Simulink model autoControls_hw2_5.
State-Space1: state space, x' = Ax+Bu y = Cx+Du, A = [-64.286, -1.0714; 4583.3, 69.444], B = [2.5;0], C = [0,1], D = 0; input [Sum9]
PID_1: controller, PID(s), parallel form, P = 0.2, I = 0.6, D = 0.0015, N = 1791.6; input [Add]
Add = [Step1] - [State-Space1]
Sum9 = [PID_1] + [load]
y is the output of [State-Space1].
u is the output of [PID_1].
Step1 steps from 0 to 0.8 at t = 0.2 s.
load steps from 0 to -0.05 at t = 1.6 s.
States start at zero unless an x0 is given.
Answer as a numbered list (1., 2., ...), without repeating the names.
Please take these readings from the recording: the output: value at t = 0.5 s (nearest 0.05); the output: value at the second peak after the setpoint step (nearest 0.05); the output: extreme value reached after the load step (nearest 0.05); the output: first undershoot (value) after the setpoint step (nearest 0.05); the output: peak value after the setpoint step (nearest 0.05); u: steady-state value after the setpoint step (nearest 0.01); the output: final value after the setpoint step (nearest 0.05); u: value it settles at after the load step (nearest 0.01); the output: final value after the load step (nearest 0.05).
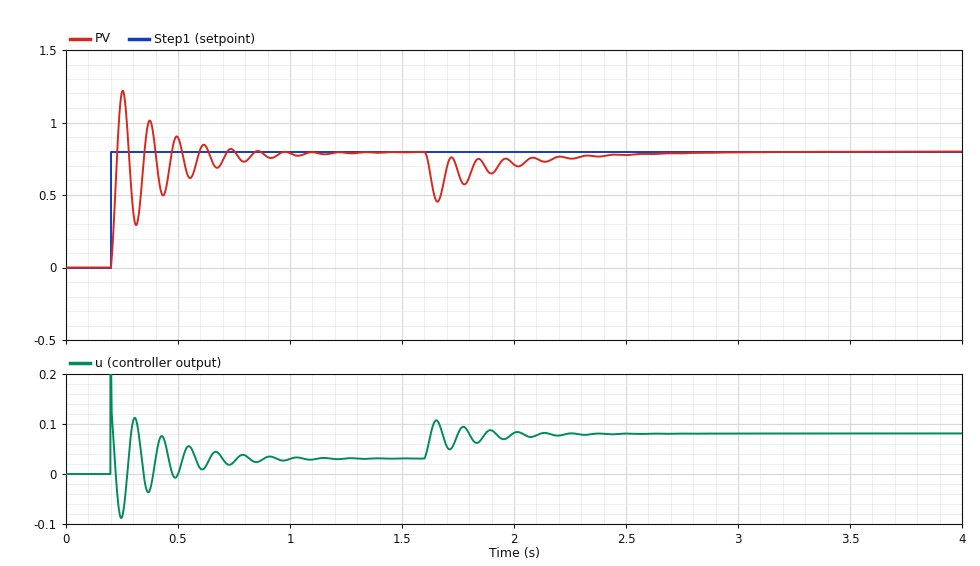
1. 0.90
2. 1.00
3. 0.45
4. 0.30
5. 1.20
6. 0.03
7. 0.80
8. 0.08
9. 0.80
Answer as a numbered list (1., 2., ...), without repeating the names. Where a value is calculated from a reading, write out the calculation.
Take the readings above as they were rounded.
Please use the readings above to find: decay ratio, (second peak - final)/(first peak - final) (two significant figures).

1. (1 - 0.8) / (1.2 - 0.8) = 0.50
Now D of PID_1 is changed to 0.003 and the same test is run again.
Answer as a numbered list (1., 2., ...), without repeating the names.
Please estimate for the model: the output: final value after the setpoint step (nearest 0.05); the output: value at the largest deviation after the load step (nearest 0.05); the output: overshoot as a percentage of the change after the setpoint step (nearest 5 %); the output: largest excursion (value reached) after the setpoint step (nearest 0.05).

1. 0.80
2. 0.50
3. 35 %
4. 1.05
